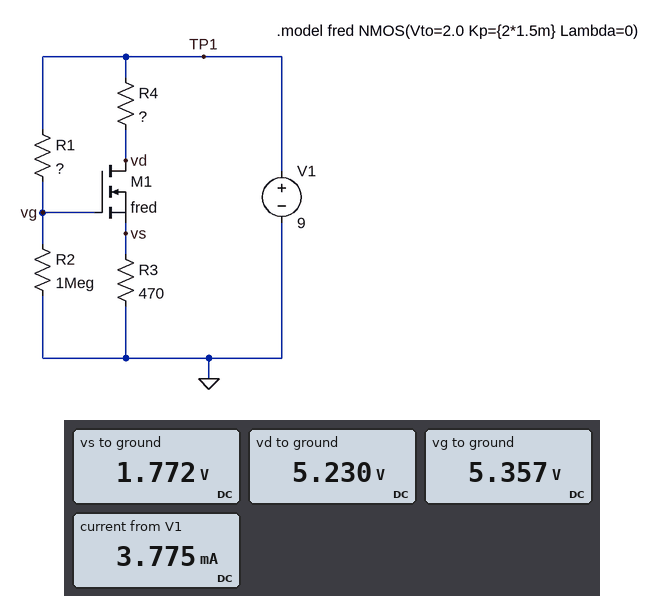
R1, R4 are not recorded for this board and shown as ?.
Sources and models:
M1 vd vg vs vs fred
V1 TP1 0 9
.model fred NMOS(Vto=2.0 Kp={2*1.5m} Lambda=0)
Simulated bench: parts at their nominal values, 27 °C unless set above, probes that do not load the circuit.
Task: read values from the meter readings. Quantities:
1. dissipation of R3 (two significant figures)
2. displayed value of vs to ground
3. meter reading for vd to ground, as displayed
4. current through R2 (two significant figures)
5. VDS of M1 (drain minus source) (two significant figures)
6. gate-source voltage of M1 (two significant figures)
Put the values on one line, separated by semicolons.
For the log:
6.7 mW; 1.772 V; 5.230 V; 5.4 µA; 3.5 V; 3.6 V
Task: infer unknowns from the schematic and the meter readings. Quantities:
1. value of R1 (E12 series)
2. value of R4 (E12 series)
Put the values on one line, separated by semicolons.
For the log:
680 kΩ; 1 kΩ
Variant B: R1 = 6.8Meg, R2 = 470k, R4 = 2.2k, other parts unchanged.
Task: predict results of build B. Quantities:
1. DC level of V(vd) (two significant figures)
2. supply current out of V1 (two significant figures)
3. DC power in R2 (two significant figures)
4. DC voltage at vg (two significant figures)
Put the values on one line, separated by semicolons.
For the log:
9.0 V; 1.2 µA; 720 nW; 580 mV
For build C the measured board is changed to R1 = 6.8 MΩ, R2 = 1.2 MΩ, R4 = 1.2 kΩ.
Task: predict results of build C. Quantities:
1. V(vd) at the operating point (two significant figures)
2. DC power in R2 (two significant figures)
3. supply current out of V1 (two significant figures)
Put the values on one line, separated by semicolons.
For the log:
9.0 V; 1.5 µW; 1.1 µA
